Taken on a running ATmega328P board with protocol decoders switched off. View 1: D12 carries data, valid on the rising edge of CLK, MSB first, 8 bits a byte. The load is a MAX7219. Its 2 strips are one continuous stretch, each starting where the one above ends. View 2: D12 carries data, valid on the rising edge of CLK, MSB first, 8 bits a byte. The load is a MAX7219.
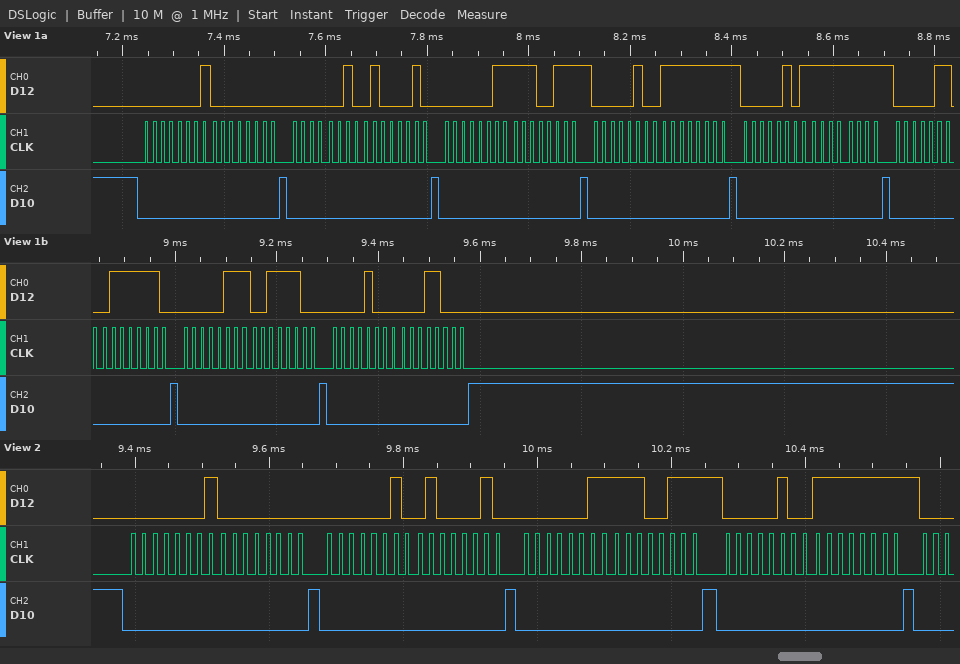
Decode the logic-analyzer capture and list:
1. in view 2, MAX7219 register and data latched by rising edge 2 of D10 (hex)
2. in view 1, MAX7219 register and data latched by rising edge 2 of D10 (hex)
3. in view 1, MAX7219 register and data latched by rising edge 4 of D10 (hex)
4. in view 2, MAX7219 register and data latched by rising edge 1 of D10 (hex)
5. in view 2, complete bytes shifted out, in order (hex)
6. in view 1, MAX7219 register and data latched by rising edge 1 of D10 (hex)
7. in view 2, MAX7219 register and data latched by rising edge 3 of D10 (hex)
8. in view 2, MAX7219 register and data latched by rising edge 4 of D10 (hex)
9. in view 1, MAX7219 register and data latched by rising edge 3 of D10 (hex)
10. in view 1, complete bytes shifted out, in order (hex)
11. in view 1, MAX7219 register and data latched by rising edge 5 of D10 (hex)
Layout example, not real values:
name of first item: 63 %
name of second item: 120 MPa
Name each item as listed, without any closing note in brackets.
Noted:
in view 2, MAX7219 register and data latched by rising edge 2 of D10: register 0x2, data 0x42
in view 1, MAX7219 register and data latched by rising edge 2 of D10: register 0x2, data 0x42
in view 1, MAX7219 register and data latched by rising edge 4 of D10: register 0x4, data 0xFF
in view 2, MAX7219 register and data latched by rising edge 1 of D10: register 0x1, data 0x00
in view 2, complete bytes shifted out, in order: 01 00 02 42 03 E7 04 FF
in view 1, MAX7219 register and data latched by rising edge 1 of D10: register 0x1, data 0x00
in view 2, MAX7219 register and data latched by rising edge 3 of D10: register 0x3, data 0xE7
in view 2, MAX7219 register and data latched by rising edge 4 of D10: register 0x4, data 0xFF
in view 1, MAX7219 register and data latched by rising edge 3 of D10: register 0x3, data 0xE7
in view 1, complete bytes shifted out, in order: 01 00 02 42 03 E7 04 FF 05 FF 06 7E 07 3C 08 18
in view 1, MAX7219 register and data latched by rising edge 5 of D10: register 0x5, data 0xFF
